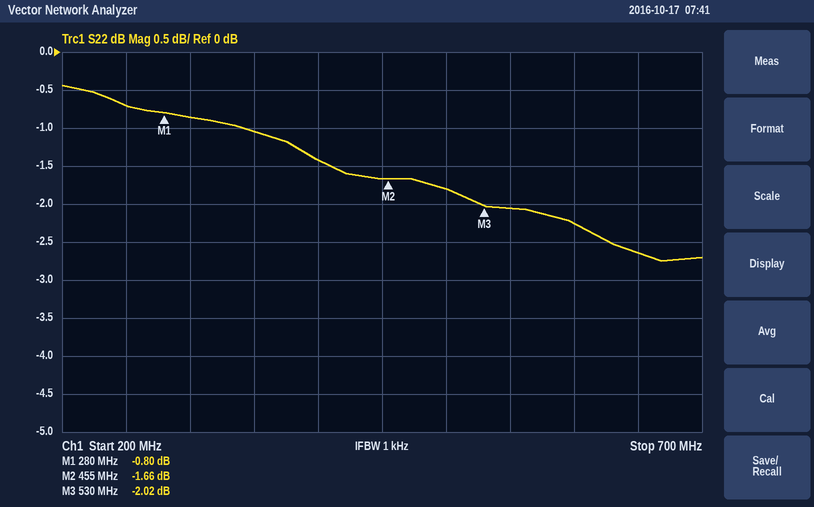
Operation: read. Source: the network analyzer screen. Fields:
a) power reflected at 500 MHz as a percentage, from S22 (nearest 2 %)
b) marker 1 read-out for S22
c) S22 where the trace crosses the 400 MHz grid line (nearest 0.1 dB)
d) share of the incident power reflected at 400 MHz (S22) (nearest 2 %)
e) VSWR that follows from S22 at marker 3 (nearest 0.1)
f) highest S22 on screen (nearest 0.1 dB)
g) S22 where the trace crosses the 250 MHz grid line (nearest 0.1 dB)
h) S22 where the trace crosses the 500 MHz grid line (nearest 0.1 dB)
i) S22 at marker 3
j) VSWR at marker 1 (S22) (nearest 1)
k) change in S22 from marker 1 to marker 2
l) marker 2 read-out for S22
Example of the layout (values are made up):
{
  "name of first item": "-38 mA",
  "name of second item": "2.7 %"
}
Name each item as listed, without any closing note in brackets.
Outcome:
{
  "power reflected at 500 MHz as a percentage, from S22": "66 %",
  "marker 1 read-out for S22": "-0.80 dB",
  "S22 where the trace crosses the 400 MHz grid line": "-1.4 dB",
  "share of the incident power reflected at 400 MHz (S22)": "72 %",
  "VSWR that follows from S22 at marker 3": "8.6",
  "highest S22 on screen": "-0.4 dB",
  "S22 where the trace crosses the 250 MHz grid line": "-0.7 dB",
  "S22 where the trace crosses the 500 MHz grid line": "-1.8 dB",
  "S22 at marker 3": "-2.02 dB",
  "VSWR at marker 1 (S22)": "22",
  "change in S22 from marker 1 to marker 2": "-0.86 dB",
  "marker 2 read-out for S22": "-1.66 dB"
}
